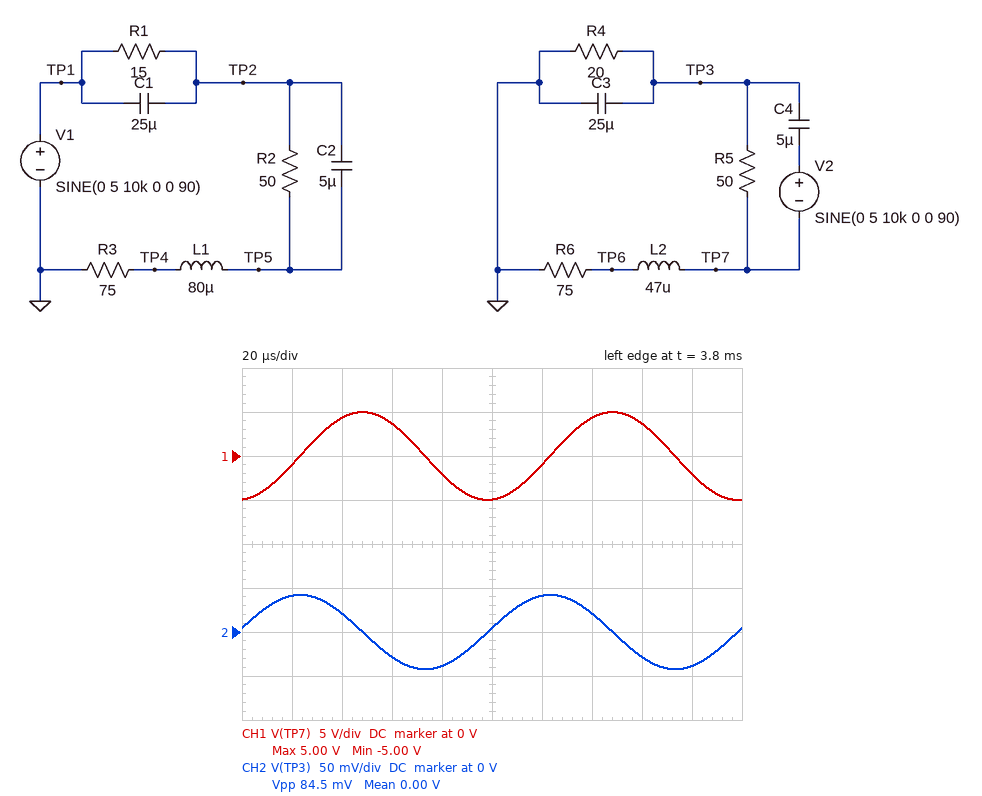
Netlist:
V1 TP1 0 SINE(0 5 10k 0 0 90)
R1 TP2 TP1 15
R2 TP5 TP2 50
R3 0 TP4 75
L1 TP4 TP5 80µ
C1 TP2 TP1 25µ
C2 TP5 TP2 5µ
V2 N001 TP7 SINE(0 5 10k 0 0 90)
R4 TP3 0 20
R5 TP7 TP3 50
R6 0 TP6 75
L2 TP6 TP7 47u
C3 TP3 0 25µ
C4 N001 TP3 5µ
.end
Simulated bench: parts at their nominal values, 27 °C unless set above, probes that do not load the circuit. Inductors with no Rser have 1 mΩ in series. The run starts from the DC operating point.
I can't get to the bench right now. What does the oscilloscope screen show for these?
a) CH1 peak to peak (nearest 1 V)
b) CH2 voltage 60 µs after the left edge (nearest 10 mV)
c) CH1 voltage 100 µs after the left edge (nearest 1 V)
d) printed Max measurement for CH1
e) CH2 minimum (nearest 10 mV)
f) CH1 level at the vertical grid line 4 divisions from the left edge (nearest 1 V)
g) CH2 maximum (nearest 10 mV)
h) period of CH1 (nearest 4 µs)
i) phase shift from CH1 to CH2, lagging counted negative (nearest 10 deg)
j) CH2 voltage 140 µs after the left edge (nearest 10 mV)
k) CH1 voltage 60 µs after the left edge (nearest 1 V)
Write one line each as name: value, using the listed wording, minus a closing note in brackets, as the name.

CH1 peak to peak: 10 V
CH2 voltage 60 µs after the left edge: -30 mV
CH1 voltage 100 µs after the left edge: -5 V
printed Max measurement for CH1: 5.00 V
CH2 minimum: -40 mV
CH1 level at the vertical grid line 4 divisions from the left edge: -2 V
CH2 maximum: 40 mV
period of CH1: 100 µs
phase shift from CH1 to CH2, lagging counted negative: 90 deg
CH2 voltage 140 µs after the left edge: 20 mV
CH1 voltage 60 µs after the left edge: 4 V
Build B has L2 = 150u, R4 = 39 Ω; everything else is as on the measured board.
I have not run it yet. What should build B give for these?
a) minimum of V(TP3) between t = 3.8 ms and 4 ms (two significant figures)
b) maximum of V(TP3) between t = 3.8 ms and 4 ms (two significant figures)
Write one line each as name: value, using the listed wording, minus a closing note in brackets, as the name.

minimum of V(TP3) between t = 3.8 ms and 4 ms: -45 mV
maximum of V(TP3) between t = 3.8 ms and 4 ms: 39 mV
